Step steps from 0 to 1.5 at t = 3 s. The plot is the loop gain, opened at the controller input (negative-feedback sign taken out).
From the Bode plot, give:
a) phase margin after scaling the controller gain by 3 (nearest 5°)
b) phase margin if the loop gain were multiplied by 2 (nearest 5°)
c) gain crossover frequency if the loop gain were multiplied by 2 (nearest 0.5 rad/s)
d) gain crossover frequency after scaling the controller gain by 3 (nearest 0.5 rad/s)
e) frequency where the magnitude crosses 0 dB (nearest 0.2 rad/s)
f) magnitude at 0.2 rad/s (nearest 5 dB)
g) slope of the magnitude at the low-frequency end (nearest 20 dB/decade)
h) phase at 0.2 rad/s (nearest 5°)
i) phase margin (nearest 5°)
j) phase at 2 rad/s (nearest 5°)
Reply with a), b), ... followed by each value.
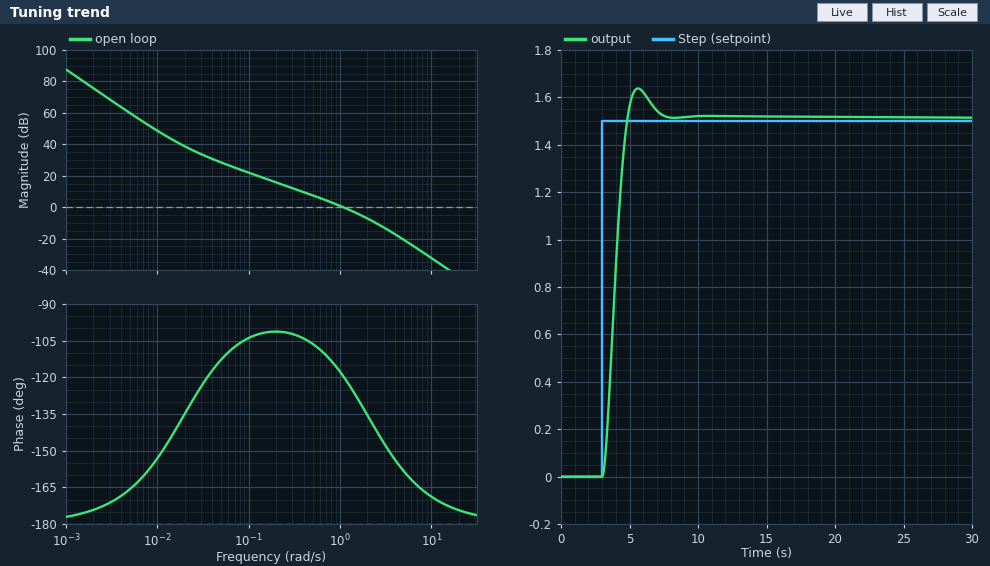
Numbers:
a) 40°
b) 45°
c) 2.0 rad/s
d) 2.5 rad/s
e) 1.0 rad/s
f) 15 dB
g) -40 dB/decade
h) -100°
i) 60°
j) -135°
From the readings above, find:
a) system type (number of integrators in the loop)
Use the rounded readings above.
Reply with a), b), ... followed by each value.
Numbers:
a) 2
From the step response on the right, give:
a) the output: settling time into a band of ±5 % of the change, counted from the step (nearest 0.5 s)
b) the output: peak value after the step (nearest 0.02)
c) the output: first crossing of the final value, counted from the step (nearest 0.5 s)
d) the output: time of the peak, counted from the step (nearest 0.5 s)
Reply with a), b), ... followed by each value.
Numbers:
a) 3.5 s
b) 1.64
c) 2.0 s
d) 2.5 s
